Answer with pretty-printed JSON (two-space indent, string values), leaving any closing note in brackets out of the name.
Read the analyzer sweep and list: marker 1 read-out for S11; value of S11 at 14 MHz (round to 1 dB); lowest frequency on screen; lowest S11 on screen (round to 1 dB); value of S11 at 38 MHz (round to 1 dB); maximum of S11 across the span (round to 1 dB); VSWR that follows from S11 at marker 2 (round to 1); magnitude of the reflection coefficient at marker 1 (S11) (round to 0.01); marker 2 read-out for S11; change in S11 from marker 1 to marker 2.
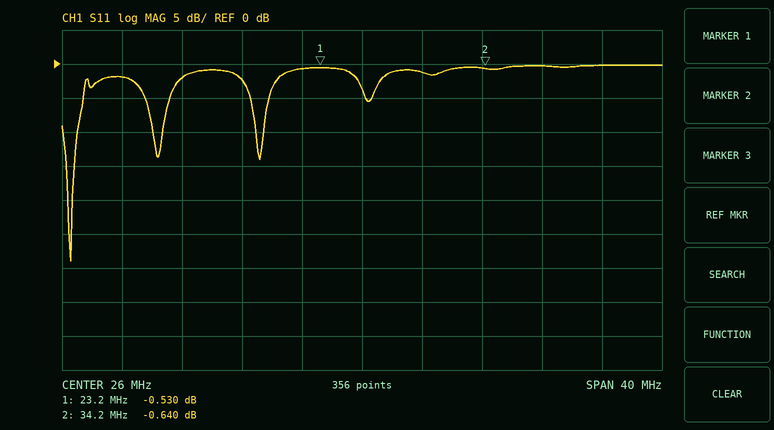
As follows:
{
  "marker 1 read-out for S11": "-0.530 dB",
  "value of S11 at 14 MHz": "-2 dB",
  "lowest frequency on screen": "6 MHz",
  "lowest S11 on screen": "-29 dB",
  "value of S11 at 38 MHz": "0 dB",
  "maximum of S11 across the span": "0 dB",
  "VSWR that follows from S11 at marker 2": "27",
  "magnitude of the reflection coefficient at marker 1 (S11)": "0.94",
  "marker 2 read-out for S11": "-0.640 dB",
  "change in S11 from marker 1 to marker 2": "-0.110 dB"
}
